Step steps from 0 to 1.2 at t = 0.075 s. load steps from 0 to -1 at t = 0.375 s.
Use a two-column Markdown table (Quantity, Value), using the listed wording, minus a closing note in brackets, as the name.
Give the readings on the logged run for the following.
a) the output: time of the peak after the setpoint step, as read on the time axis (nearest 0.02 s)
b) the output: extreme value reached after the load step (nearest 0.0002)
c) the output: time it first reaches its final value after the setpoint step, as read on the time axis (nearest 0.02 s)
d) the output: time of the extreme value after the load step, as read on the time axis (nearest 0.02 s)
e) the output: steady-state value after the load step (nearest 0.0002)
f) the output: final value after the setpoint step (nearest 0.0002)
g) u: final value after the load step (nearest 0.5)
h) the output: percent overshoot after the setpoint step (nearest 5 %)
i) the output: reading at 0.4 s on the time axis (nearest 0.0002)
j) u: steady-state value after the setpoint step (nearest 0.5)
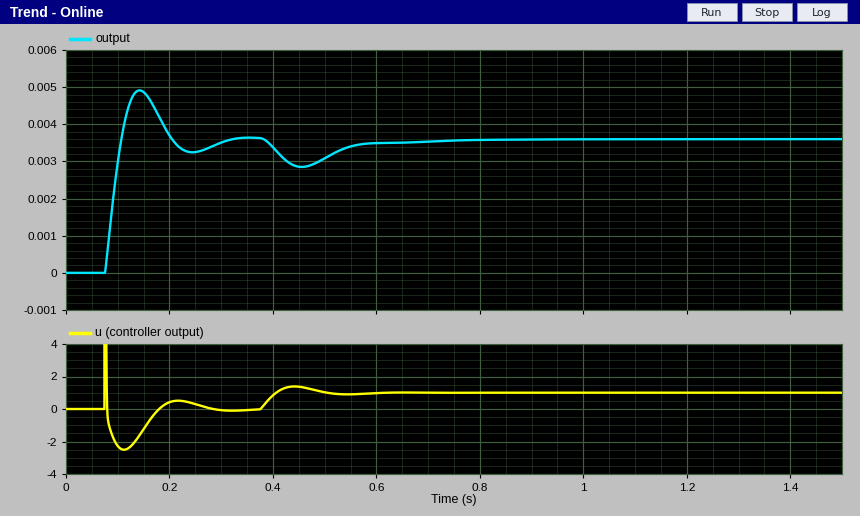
| Quantity | Value |
|---|---|
| the output: time of the peak after the setpoint step, as read on the time axis | 0.14 s |
| the output: extreme value reached after the load step | 0.0028 |
| the output: time it first reaches its final value after the setpoint step, as read on the time axis | 0.10 s |
| the output: time of the extreme value after the load step, as read on the time axis | 0.46 s |
| the output: steady-state value after the load step | 0.0036 |
| the output: final value after the setpoint step | 0.0036 |
| u: final value after the load step | 1.0 |
| the output: percent overshoot after the setpoint step | 35 % |
| the output: reading at 0.4 s on the time axis | 0.0034 |
| u: steady-state value after the setpoint step | 0.0 |
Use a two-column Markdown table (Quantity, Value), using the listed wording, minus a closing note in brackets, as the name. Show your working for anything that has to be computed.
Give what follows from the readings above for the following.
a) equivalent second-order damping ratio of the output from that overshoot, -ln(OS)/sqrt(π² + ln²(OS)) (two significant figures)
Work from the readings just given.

| Quantity | Value |
|---|---|
| equivalent second-order damping ratio of the output from that overshoot, -ln(OS)/sqrt(π² + ln²(OS)) | ln(0.35) = -1.050; 1.050 / sqrt(9.870 + 1.102) = 0.32 |
